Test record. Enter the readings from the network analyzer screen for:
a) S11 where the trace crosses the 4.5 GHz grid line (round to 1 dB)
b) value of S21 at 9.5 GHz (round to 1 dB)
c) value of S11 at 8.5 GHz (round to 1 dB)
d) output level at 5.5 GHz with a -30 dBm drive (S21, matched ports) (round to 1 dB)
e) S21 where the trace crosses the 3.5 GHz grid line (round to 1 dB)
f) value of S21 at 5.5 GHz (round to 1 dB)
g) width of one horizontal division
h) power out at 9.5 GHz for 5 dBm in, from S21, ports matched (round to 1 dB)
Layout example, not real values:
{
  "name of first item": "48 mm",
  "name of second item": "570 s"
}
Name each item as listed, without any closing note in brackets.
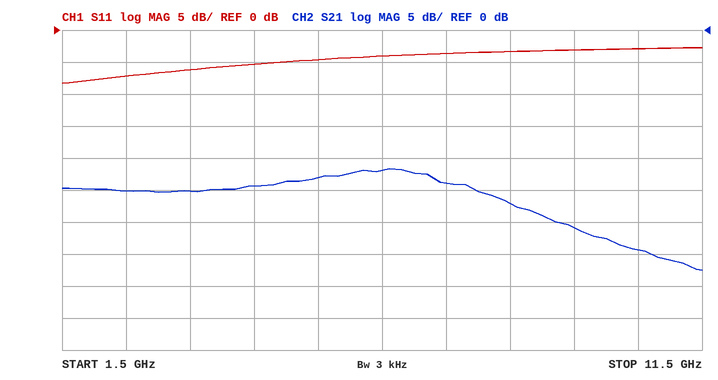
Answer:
{
  "S11 where the trace crosses the 4.5 GHz grid line": "-5 dB",
  "value of S21 at 9.5 GHz": "-31 dB",
  "value of S11 at 8.5 GHz": "-3 dB",
  "output level at 5.5 GHz with a -30 dBm drive (S21, matched ports)": "-53 dBm",
  "S21 where the trace crosses the 3.5 GHz grid line": "-25 dB",
  "value of S21 at 5.5 GHz": "-23 dB",
  "width of one horizontal division": "1 GHz",
  "power out at 9.5 GHz for 5 dBm in, from S21, ports matched": "-26 dBm"
}
